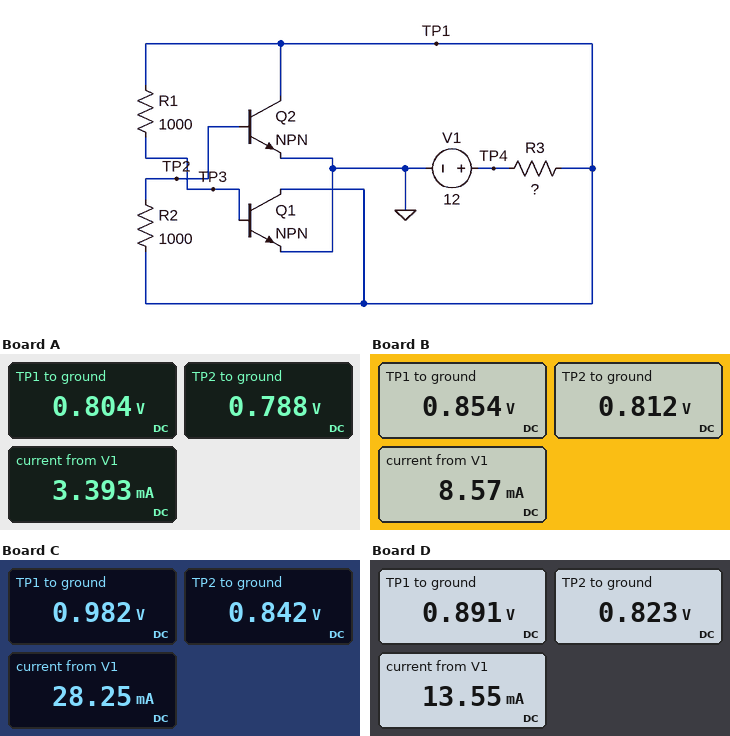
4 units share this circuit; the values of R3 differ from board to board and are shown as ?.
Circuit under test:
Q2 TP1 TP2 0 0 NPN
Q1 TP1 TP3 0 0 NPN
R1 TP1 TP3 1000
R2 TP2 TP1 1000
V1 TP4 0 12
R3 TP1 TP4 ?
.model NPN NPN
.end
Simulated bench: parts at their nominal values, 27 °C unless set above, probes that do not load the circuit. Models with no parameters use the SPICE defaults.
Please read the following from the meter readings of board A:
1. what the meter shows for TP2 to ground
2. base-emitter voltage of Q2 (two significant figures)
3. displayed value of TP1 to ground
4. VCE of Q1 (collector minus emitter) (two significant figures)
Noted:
0.788 V
790 mV
0.804 V
800 mV
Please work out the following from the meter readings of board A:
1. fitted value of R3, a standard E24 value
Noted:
3.3 kΩ
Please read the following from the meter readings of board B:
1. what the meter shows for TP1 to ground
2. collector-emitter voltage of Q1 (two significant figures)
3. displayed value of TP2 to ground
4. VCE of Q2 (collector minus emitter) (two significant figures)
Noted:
0.854 V
850 mV
0.812 V
850 mV
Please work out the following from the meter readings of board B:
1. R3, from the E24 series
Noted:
1.3 kΩ
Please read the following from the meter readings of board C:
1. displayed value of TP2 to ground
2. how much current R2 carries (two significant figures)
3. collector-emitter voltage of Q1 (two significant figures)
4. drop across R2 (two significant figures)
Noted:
0.842 V
140 µA
980 mV
140 mV
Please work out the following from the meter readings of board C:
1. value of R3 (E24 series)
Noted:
390 Ω
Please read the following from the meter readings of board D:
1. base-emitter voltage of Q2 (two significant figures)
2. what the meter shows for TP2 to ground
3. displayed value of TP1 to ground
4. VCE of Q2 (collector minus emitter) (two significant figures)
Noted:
820 mV
0.823 V
0.891 V
890 mV
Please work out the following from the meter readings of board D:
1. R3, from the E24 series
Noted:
820 Ω
